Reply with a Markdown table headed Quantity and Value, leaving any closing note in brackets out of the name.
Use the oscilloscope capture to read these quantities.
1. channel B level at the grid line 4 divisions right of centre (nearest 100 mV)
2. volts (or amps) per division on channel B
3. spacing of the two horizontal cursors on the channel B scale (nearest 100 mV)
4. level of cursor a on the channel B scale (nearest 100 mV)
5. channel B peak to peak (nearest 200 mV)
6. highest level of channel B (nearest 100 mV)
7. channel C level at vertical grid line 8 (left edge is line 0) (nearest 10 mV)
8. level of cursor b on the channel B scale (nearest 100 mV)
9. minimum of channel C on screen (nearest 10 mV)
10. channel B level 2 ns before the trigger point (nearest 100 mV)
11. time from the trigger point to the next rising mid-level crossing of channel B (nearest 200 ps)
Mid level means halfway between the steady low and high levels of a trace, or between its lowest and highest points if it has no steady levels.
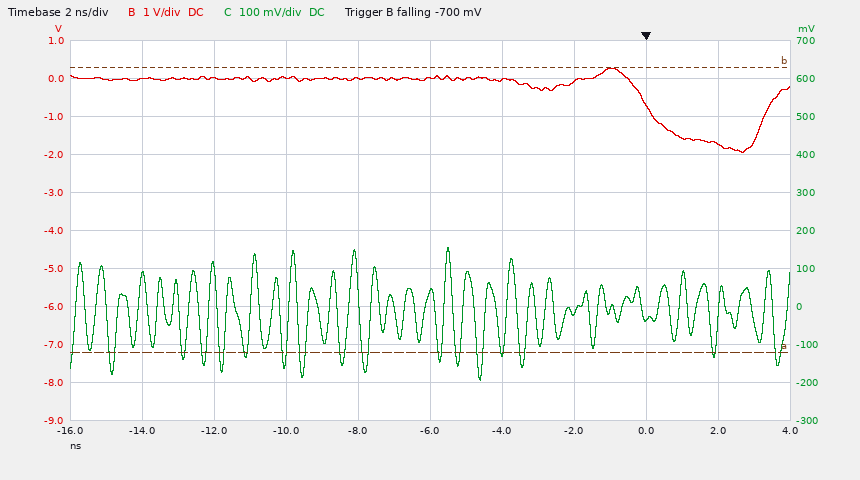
| Quantity | Value |
|---|---|
| channel B level at the grid line 4 divisions right of centre | -1.7 V |
| volts (or amps) per division on channel B | 1 V |
| spacing of the two horizontal cursors on the channel B scale | 7.5 V |
| level of cursor a on the channel B scale | -7.2 V |
| channel B peak to peak | 2.2 V |
| highest level of channel B | 300 mV |
| channel C level at vertical grid line 8 (left edge is line 0) | -30 mV |
| level of cursor b on the channel B scale | 300 mV |
| minimum of channel C on screen | -190 mV |
| channel B level 2 ns before the trigger point | -100 mV |
| time from the trigger point to the next rising mid-level crossing of channel B | 3.4 ns |
